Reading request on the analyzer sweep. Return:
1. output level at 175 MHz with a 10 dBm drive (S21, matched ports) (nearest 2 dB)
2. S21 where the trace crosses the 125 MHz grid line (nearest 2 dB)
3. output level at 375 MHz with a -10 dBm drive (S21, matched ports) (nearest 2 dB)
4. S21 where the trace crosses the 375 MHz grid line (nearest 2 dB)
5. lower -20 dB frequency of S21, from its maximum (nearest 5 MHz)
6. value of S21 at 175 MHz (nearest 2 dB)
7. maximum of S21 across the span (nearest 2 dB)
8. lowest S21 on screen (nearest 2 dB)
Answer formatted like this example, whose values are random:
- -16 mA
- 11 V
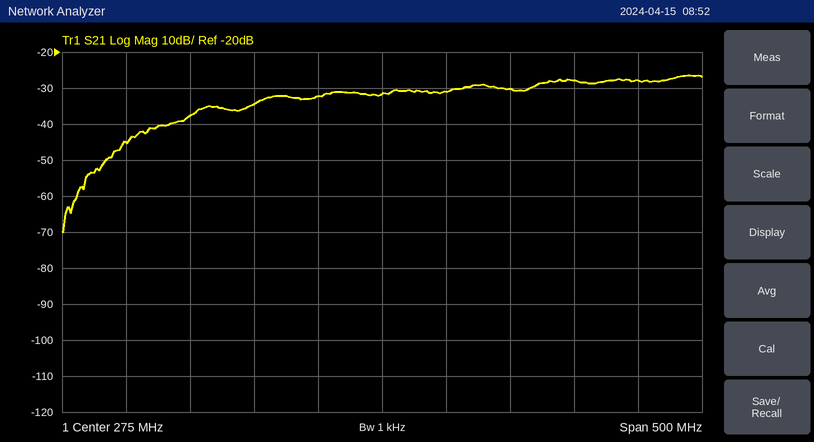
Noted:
- -24 dBm
- -38 dB
- -40 dBm
- -30 dB
- 70 MHz
- -34 dB
- -26 dB
- -70 dB
